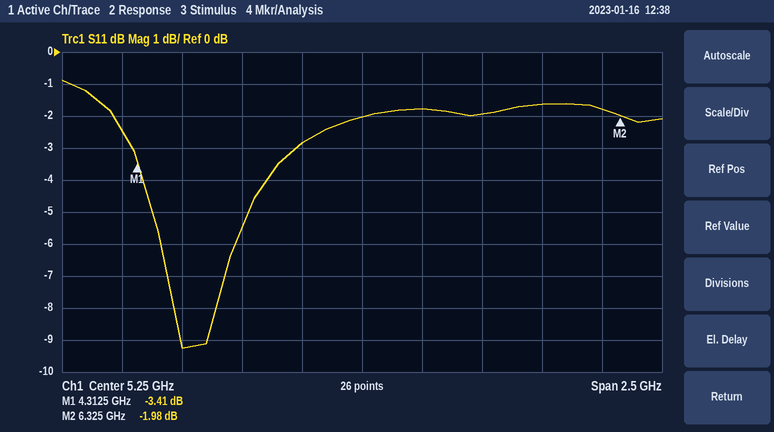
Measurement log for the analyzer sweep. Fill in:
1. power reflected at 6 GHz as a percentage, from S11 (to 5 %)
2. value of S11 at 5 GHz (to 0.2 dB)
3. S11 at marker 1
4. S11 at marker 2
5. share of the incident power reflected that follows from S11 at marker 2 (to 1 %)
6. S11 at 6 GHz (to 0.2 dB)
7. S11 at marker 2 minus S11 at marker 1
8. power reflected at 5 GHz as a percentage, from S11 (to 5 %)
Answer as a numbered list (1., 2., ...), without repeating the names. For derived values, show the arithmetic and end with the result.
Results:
1. 10^(-1.6/10) ≈ 69.2 %, so 70 % to the nearest 5 %
2. -2.8 dB
3. -3.41 dB
4. -1.98 dB
5. 10^(-1.98/10) ≈ 63 %
6. -1.6 dB
7. -1.98 − (-3.41) = 1.43 dB
8. 10^(-2.8/10) ≈ 52.5 %, so 50 % to the nearest 5 %
